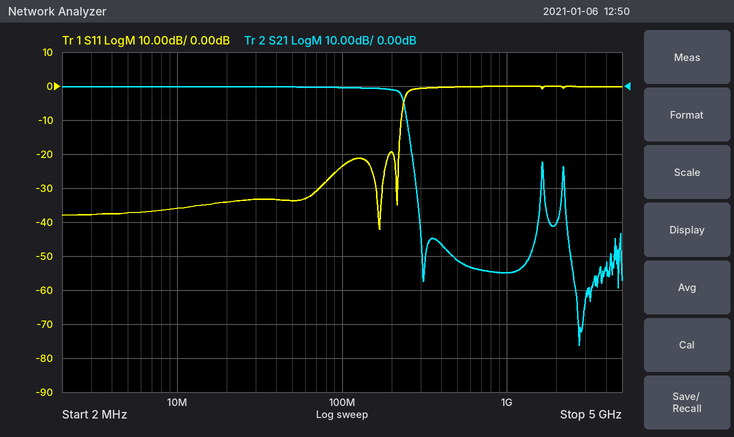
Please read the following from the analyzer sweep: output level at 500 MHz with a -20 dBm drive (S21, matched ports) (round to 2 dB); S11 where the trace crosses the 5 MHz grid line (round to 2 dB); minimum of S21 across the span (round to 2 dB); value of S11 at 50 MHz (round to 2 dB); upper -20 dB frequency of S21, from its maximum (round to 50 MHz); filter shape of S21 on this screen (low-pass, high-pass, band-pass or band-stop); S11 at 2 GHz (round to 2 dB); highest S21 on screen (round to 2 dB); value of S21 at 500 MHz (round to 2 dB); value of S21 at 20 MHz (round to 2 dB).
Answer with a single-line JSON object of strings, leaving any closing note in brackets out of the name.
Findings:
{"output level at 500 MHz with a -20 dBm drive (S21, matched ports)": "-72 dBm", "S11 where the trace crosses the 5 MHz grid line": "-38 dB", "minimum of S21 across the span": "-76 dB", "value of S11 at 50 MHz": "-34 dB", "upper -20 dB frequency of S21, from its maximum": "250 MHz", "filter shape of S21 on this screen": "low-pass", "S11 at 2 GHz": "0 dB", "highest S21 on screen": "0 dB", "value of S21 at 500 MHz": "-52 dB", "value of S21 at 20 MHz": "0 dB"}
